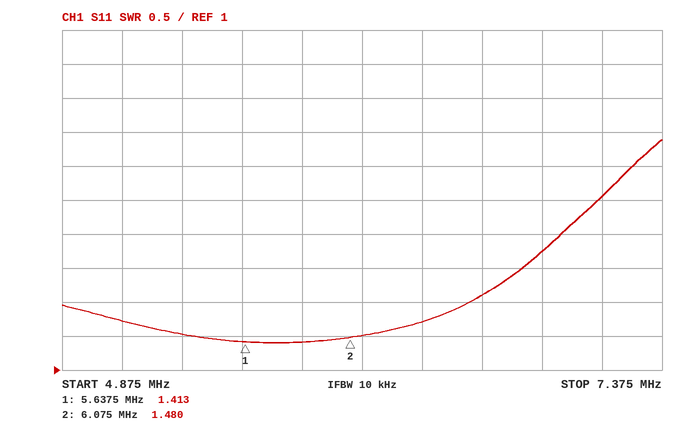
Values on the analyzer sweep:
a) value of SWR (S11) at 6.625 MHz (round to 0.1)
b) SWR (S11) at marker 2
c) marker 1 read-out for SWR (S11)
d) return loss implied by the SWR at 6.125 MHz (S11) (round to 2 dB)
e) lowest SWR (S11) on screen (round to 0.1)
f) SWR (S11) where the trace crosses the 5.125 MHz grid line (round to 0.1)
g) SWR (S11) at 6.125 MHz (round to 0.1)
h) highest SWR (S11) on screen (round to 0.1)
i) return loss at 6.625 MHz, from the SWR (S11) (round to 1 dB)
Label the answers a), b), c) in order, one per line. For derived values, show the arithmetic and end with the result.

a) 2.1
b) 1.480
c) 1.413
d) −20 log10((1.5 − 1)/(1.5 + 1)) ≈ 14 dB
e) 1.4
f) 1.7
g) 1.5
h) 4.4
i) −20 log10((2.1 − 1)/(2.1 + 1)) ≈ 9 dB
